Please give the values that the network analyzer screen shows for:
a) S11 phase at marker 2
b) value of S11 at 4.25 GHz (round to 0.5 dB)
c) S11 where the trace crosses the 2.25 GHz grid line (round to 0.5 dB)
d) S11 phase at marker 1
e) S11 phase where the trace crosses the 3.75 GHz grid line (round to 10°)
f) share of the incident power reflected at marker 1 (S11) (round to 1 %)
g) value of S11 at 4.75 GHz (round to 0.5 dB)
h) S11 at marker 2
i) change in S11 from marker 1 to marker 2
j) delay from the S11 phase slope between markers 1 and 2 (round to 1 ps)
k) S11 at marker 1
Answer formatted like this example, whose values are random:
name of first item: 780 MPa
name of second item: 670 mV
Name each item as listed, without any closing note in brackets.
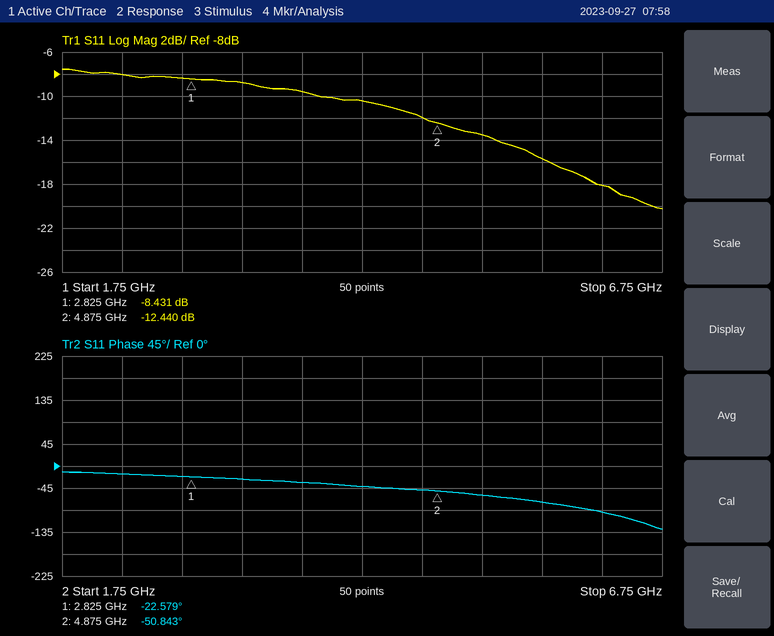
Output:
S11 phase at marker 2: -50.843°
value of S11 at 4.25 GHz: -10.5 dB
S11 where the trace crosses the 2.25 GHz grid line: -8.0 dB
S11 phase at marker 1: -22.579°
S11 phase where the trace crosses the 3.75 GHz grid line: -30°
share of the incident power reflected at marker 1 (S11): 14 %
value of S11 at 4.75 GHz: -12.0 dB
S11 at marker 2: -12.440 dB
change in S11 from marker 1 to marker 2: -4.009 dB
delay from the S11 phase slope between markers 1 and 2: 38 ps
S11 at marker 1: -8.431 dB
